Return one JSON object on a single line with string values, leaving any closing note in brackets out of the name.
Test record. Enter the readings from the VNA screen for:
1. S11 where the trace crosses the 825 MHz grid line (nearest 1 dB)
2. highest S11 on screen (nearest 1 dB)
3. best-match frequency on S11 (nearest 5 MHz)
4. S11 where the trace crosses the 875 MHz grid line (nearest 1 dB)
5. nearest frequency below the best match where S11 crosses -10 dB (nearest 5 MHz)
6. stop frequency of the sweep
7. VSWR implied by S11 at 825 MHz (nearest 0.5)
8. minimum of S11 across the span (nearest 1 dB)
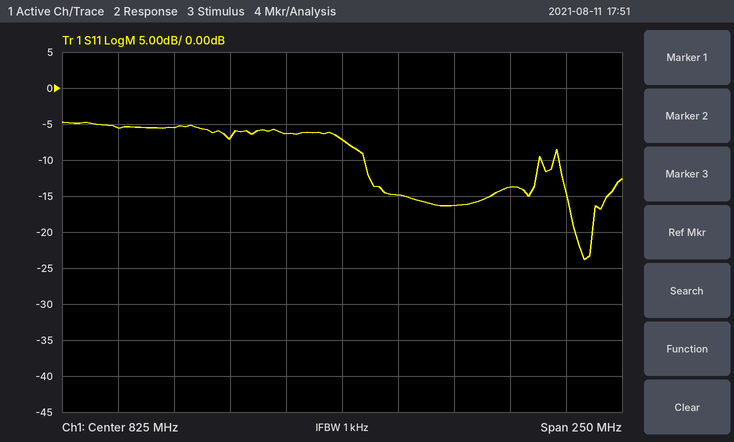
{"S11 where the trace crosses the 825 MHz grid line": "-7 dB", "highest S11 on screen": "-5 dB", "best-match frequency on S11": "935 MHz", "S11 where the trace crosses the 875 MHz grid line": "-16 dB", "nearest frequency below the best match where S11 crosses -10 dB": "920 MHz", "stop frequency of the sweep": "950 MHz", "VSWR implied by S11 at 825 MHz": "2.5", "minimum of S11 across the span": "-24 dB"}
